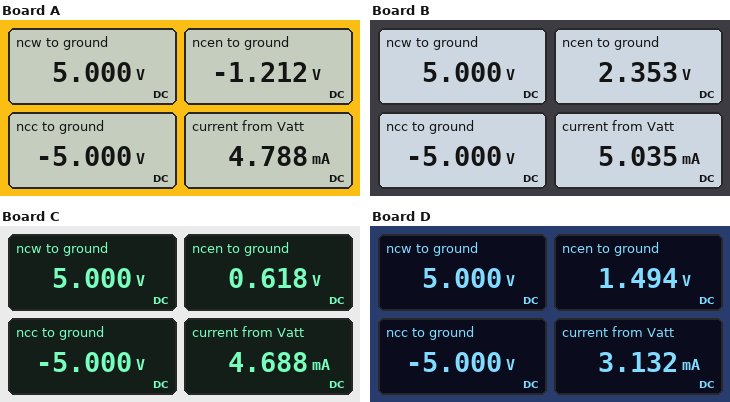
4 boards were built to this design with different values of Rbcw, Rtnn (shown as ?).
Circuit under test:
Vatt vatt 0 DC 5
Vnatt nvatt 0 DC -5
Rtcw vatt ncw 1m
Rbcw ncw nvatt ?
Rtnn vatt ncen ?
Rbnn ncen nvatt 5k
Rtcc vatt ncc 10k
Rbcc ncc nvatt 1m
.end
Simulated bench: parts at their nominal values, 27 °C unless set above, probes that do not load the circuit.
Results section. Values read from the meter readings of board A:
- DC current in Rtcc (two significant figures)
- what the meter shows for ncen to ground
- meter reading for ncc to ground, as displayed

1.0 mA
-1.212 V
-5.000 V
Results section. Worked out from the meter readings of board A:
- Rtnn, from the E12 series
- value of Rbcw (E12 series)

8.2 kΩ
3.3 kΩ
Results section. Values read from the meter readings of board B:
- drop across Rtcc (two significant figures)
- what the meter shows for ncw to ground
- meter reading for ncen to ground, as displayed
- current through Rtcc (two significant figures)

10 V
5.000 V
2.353 V
1.0 mA
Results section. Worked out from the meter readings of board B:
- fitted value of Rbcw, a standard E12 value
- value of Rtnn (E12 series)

3.9 kΩ
1.8 kΩ
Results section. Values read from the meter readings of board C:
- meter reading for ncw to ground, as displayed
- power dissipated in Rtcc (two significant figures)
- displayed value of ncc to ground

5.000 V
10 mW
-5.000 V
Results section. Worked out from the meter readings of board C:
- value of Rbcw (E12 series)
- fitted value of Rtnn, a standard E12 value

3.9 kΩ
3.9 kΩ
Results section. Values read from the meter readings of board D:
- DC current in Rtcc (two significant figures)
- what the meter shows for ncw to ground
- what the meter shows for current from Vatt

1.0 mA
5.000 V
3.132 mA
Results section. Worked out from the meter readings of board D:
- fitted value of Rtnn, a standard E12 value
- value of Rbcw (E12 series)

2.7 kΩ
12 kΩ
